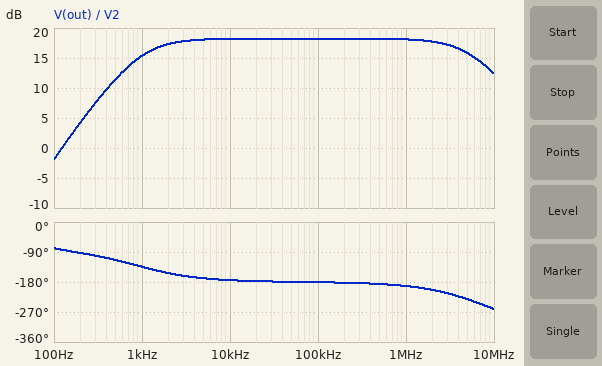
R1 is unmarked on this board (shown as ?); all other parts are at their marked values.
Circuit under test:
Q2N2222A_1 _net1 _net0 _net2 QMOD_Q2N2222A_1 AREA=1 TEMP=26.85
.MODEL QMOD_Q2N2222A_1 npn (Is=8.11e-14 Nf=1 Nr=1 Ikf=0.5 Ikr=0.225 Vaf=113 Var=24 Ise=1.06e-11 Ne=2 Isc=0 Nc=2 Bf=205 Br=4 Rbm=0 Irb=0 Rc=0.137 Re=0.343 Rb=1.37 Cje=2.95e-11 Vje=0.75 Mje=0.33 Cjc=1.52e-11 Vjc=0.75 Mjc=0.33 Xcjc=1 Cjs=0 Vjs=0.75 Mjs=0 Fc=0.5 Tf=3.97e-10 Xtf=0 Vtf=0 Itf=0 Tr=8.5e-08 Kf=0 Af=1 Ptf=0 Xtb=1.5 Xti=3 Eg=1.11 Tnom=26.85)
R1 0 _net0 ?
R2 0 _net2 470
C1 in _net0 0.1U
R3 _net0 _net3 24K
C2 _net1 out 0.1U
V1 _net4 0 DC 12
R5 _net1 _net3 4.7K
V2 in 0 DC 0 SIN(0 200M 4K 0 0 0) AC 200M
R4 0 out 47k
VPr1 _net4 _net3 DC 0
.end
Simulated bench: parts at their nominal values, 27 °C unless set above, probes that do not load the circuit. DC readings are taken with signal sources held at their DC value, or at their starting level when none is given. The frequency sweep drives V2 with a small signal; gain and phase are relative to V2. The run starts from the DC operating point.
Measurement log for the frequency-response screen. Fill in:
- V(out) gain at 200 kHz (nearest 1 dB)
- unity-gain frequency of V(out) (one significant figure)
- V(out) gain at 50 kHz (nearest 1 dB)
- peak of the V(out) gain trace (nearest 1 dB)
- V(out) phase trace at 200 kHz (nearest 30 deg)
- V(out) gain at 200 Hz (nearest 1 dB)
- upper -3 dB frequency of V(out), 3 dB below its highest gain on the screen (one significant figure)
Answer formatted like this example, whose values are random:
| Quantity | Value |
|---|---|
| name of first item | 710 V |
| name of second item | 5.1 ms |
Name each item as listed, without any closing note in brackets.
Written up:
| Quantity | Value |
|---|---|
| V(out) gain at 200 kHz | 18 dB |
| unity-gain frequency of V(out) | 100 Hz |
| V(out) gain at 50 kHz | 18 dB |
| peak of the V(out) gain trace | 18 dB |
| V(out) phase trace at 200 kHz | -180 deg |
| V(out) gain at 200 Hz | 4 dB |
| upper -3 dB frequency of V(out), 3 dB below its highest gain on the screen | 6 MHz |
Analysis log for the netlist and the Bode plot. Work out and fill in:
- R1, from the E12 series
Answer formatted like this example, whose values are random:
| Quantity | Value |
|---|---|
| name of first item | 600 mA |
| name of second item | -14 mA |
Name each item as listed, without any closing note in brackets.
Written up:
| Quantity | Value |
|---|---|
| R1, from the E12 series | 1.8 kΩ |
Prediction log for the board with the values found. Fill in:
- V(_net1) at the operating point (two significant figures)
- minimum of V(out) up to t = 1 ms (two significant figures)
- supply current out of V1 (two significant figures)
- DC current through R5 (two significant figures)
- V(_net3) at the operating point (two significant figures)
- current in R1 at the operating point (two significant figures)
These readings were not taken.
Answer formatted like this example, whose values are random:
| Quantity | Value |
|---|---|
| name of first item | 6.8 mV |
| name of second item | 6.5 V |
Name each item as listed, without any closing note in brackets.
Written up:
| Quantity | Value |
|---|---|
| V(_net1) at the operating point | 9.5 V |
| minimum of V(out) up to t = 1 ms | -1.6 V |
| supply current out of V1 | 990 µA |
| DC current through R5 | 530 µA |
| V(_net3) at the operating point | 12 V |
| current in R1 at the operating point | 460 µA |
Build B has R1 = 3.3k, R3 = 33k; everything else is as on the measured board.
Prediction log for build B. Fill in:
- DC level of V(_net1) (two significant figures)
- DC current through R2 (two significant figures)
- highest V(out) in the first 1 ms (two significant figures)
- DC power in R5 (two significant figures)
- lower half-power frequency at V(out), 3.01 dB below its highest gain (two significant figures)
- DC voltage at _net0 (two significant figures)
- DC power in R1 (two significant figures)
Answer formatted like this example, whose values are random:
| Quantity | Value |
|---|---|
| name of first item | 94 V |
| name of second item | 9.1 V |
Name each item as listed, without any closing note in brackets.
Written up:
| Quantity | Value |
|---|---|
| DC level of V(_net1) | 7.3 V |
| DC current through R2 | 1.0 mA |
| highest V(out) in the first 1 ms | 1.8 V |
| DC power in R5 | 4.7 mW |
| lower half-power frequency at V(out), 3.01 dB below its highest gain | 550 Hz |
| DC voltage at _net0 | 1.1 V |
| DC power in R1 | 350 µW |
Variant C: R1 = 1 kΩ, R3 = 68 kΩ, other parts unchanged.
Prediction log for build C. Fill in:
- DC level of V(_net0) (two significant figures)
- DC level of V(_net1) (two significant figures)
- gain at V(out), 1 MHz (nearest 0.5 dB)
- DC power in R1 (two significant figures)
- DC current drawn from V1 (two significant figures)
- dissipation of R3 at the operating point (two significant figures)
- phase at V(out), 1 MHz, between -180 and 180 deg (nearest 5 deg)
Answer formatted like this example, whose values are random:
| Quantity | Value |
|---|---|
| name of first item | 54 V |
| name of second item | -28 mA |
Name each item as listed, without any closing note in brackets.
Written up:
| Quantity | Value |
|---|---|
| DC level of V(_net0) | 170 mV |
| DC level of V(_net1) | 12 V |
| gain at V(out), 1 MHz | -16.0 dB |
| DC power in R1 | 30 µW |
| DC current drawn from V1 | 170 µA |
| dissipation of R3 at the operating point | 2.1 mW |
| phase at V(out), 1 MHz, between -180 and 180 deg | 80 deg |
